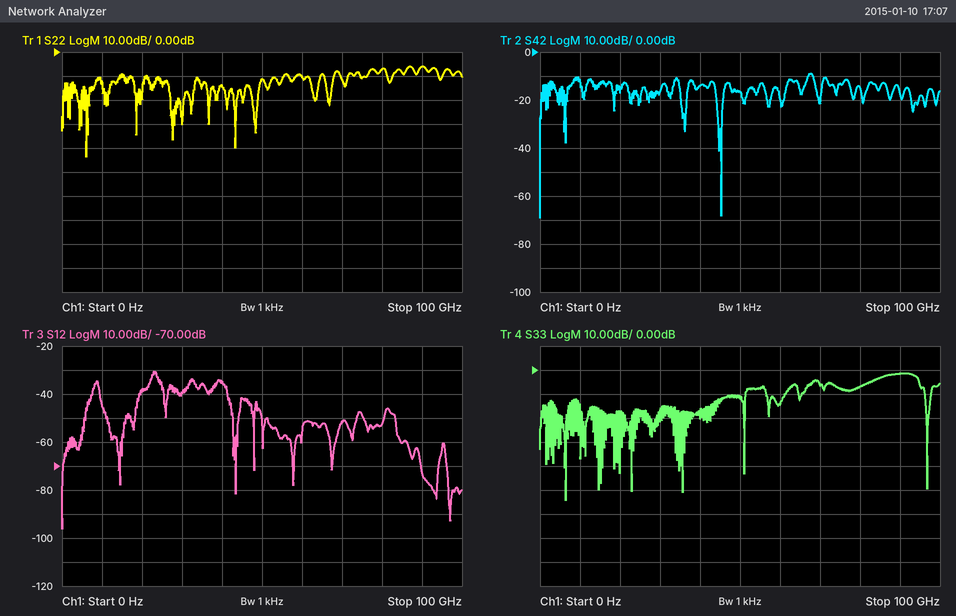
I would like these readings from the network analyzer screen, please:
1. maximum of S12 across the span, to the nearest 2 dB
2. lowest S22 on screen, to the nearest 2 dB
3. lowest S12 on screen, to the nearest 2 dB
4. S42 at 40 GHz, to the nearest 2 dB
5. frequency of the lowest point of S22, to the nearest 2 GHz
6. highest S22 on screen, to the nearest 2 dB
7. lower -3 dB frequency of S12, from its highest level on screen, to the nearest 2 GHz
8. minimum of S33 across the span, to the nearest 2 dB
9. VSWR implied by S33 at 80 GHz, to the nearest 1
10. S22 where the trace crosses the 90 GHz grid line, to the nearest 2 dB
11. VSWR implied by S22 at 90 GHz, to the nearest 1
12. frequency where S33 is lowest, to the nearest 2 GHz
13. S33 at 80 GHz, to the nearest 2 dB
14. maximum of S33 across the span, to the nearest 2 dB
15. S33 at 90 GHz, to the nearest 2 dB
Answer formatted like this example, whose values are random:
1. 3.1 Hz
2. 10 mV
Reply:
1. -30 dB
2. -44 dB
3. -96 dB
4. -14 dB
5. 6 GHz
6. -6 dB
7. 22 GHz
8. -54 dB
9. 3
10. -6 dB
11. 3
12. 6 GHz
13. -6 dB
14. -2 dB
15. -2 dB
